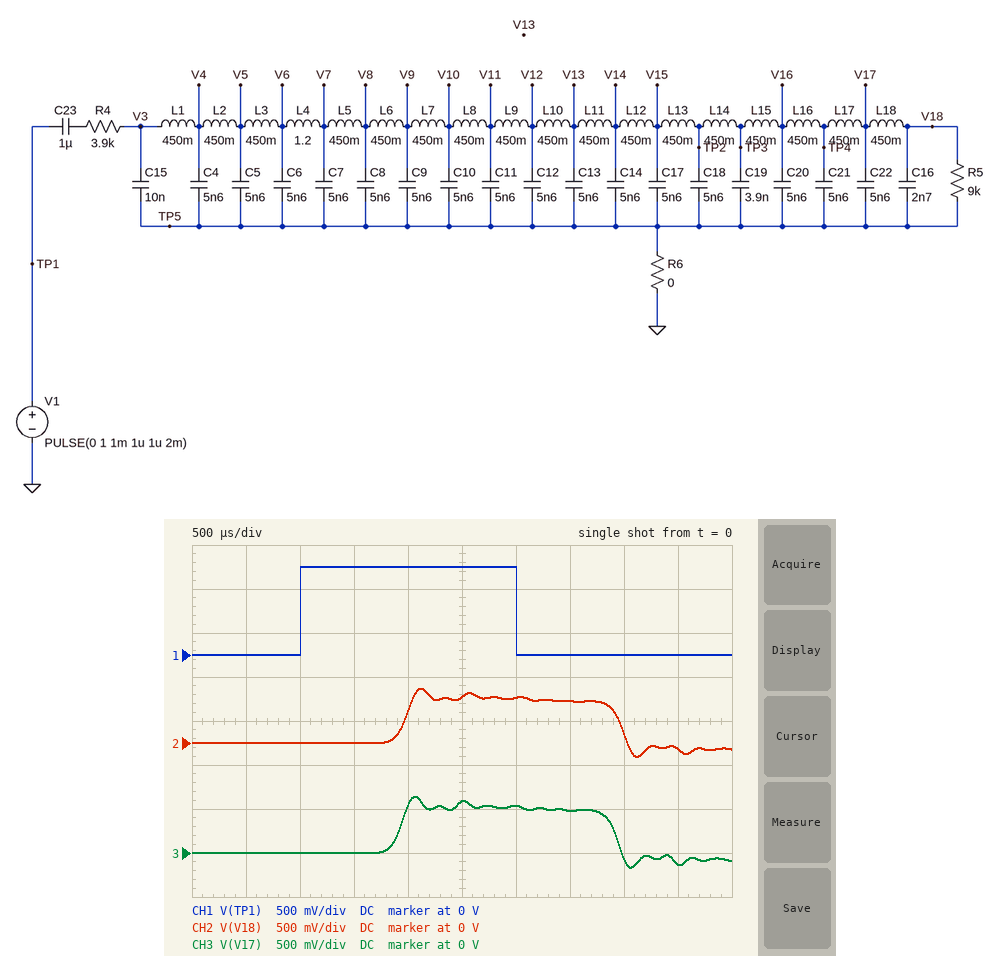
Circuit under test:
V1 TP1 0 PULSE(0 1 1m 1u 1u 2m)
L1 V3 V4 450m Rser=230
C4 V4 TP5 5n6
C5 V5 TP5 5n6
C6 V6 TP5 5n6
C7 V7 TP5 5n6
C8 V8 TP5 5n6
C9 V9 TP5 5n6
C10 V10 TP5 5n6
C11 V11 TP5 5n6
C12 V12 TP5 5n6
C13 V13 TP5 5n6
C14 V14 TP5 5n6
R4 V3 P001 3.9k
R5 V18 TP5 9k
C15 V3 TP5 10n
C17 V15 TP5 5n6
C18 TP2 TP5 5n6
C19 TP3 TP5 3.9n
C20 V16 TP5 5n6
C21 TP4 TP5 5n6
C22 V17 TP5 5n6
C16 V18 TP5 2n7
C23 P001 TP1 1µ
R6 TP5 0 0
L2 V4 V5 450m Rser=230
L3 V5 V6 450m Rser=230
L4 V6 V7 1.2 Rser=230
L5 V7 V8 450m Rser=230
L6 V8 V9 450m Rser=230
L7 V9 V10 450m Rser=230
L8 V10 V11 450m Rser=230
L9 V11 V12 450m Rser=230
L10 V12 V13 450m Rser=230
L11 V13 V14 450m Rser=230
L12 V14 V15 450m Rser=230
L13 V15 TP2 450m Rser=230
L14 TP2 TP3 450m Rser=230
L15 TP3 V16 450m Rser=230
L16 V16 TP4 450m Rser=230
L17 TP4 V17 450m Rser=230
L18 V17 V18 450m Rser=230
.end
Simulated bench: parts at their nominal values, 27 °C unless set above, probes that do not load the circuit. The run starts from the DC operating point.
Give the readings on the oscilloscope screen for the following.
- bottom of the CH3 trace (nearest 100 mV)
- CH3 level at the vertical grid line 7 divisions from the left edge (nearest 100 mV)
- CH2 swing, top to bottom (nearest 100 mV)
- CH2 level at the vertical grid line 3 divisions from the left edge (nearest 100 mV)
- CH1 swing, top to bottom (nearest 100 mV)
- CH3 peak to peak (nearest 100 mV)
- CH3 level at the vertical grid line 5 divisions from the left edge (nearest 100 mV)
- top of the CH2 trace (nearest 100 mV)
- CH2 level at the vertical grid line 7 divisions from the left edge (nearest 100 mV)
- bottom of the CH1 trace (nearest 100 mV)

-200 mV
500 mV
800 mV
0 V
1.0 V
800 mV
600 mV
600 mV
500 mV
0 V
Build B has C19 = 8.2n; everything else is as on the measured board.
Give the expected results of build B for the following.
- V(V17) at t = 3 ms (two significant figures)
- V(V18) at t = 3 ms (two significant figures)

520 mV
500 mV
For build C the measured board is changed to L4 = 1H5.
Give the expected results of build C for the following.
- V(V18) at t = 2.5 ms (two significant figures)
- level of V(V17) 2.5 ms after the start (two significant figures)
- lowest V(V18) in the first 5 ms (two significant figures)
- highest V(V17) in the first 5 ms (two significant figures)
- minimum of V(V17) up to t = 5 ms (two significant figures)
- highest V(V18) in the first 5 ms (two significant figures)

510 mV
570 mV
-130 mV
610 mV
-140 mV
590 mV
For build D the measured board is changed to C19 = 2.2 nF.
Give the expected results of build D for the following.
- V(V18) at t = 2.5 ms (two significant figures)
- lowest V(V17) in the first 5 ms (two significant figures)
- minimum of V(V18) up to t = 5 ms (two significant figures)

530 mV
-160 mV
-150 mV
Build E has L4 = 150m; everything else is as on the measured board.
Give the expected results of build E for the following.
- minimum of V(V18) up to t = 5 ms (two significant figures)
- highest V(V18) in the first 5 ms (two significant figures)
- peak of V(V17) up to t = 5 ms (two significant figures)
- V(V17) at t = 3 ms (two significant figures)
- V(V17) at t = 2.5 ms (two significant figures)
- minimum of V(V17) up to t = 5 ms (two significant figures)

-180 mV
640 mV
670 mV
520 mV
540 mV
-200 mV
